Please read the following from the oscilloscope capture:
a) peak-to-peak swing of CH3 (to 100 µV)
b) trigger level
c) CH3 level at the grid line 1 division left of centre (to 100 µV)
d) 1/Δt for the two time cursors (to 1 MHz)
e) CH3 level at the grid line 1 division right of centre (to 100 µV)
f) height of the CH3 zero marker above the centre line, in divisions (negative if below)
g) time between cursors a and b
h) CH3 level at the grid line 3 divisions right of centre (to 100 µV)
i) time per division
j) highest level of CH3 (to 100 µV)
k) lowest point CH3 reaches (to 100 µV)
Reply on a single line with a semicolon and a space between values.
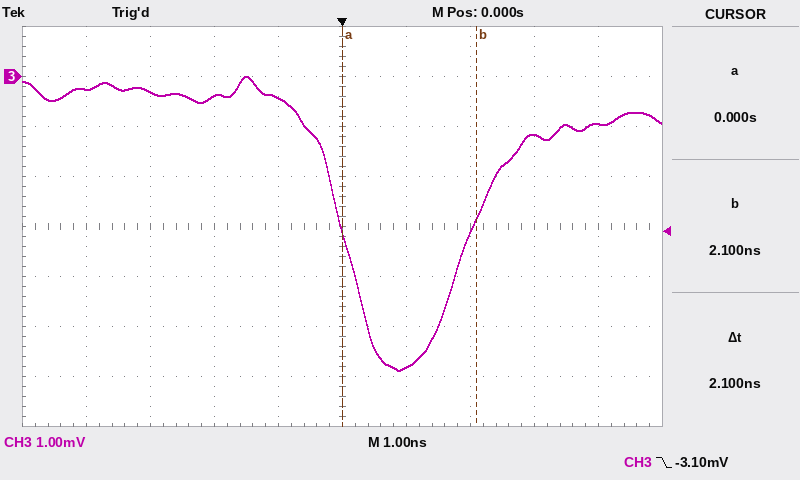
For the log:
5.9 mV; -3.10 mV; -400 µV; 476 MHz; -5.8 mV; +3.0 div; 2.1 ns; -1.2 mV; 1 ns; 0.0 mV; -5.9 mV
